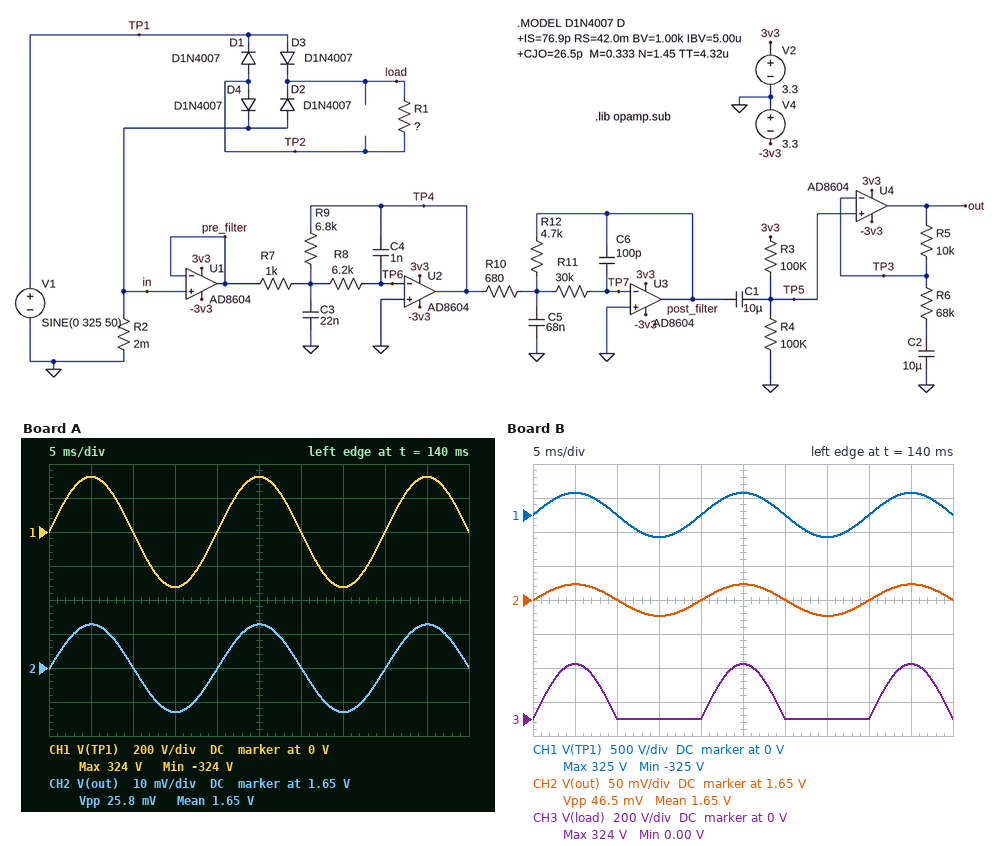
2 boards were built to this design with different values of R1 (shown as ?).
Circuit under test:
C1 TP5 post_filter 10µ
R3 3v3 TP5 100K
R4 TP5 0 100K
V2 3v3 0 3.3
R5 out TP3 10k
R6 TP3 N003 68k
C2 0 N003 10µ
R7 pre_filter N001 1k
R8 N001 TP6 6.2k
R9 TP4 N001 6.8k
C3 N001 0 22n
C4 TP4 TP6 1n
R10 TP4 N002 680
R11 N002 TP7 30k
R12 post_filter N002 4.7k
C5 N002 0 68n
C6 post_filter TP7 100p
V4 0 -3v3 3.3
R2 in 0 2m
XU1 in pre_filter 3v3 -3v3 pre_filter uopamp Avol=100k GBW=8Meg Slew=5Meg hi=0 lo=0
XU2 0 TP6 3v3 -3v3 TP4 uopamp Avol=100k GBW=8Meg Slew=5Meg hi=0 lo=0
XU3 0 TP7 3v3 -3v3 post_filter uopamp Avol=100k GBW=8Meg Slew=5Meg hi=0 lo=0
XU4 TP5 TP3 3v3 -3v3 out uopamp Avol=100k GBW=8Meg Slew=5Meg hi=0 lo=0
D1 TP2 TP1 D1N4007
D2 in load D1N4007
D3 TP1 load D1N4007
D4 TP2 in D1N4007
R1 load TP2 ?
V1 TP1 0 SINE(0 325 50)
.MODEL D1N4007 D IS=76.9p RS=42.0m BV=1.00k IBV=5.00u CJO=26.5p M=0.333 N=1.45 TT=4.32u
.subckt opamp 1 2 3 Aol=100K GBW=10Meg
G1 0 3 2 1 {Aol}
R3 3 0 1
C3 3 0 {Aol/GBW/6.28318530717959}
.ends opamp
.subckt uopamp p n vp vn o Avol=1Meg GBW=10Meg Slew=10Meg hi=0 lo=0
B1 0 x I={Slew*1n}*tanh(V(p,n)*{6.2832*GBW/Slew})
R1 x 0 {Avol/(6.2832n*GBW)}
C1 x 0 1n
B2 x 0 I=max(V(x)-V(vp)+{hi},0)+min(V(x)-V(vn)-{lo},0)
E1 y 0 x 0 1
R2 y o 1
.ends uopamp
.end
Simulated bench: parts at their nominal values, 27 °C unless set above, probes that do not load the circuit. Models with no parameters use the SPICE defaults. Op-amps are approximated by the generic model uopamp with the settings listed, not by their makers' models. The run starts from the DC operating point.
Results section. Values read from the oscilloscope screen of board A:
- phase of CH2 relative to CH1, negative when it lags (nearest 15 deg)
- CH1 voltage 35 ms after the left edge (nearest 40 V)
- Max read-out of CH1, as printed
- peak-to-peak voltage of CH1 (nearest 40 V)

0 deg
-320 V
324 V
640 V
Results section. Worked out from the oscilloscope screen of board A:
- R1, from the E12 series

2.7 kΩ
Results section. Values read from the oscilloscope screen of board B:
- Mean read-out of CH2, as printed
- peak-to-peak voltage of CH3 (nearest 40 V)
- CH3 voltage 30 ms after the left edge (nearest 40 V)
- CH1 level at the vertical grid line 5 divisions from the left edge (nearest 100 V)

1.65 V
320 V
0 V
300 V
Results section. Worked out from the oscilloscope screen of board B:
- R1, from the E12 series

1.5 kΩ
